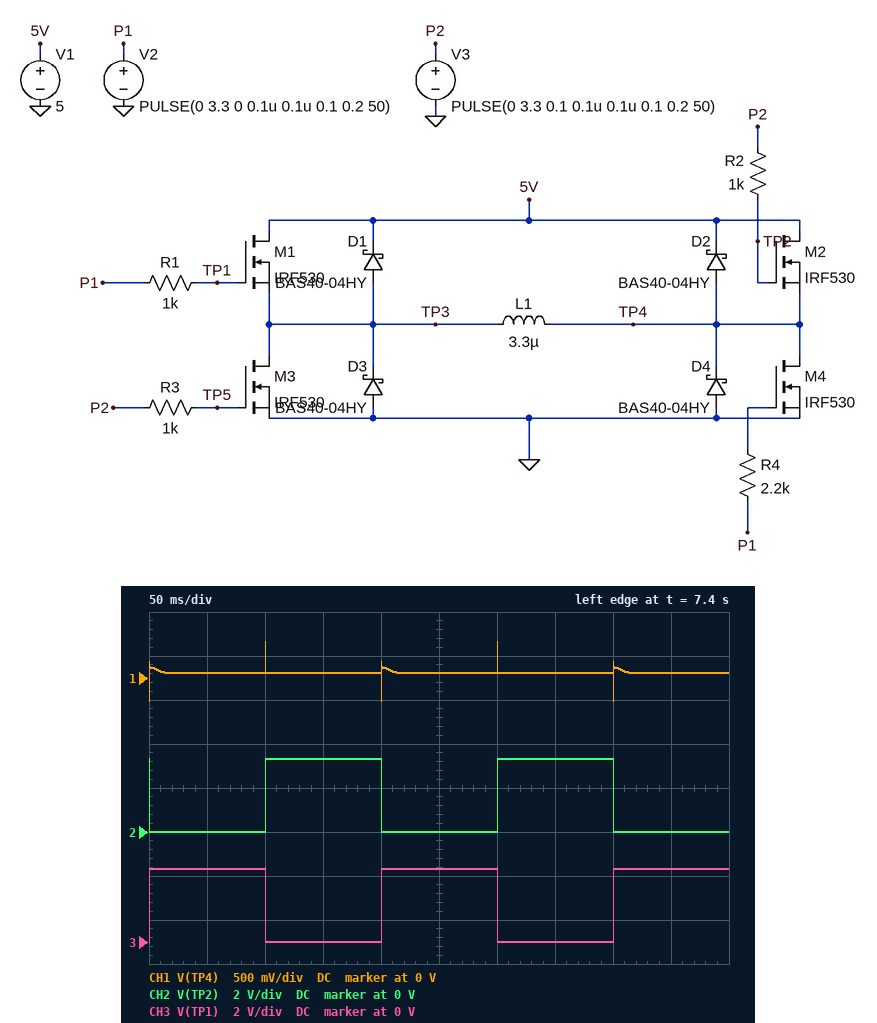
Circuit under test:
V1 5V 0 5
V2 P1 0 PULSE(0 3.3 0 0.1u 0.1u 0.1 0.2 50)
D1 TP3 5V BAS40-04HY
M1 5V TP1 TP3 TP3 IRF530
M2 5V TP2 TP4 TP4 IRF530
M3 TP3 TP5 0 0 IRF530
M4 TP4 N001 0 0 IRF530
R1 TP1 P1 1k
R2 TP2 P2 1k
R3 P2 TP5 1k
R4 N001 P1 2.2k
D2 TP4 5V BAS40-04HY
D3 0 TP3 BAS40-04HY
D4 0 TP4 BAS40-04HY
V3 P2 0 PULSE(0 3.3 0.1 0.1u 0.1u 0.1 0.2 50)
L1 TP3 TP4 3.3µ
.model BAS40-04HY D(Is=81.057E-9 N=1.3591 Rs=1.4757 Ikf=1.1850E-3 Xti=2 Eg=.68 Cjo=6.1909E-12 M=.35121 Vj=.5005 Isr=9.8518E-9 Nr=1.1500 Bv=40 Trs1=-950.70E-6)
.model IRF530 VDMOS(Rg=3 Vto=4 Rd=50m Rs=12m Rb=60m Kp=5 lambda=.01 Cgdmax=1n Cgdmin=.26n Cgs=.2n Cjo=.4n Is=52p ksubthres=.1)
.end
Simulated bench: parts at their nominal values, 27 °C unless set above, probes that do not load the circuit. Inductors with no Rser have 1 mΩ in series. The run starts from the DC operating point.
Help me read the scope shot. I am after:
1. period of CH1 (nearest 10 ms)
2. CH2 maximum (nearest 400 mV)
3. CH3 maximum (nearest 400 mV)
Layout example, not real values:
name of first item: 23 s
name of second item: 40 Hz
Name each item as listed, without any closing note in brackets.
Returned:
period of CH1: 200 ms
CH2 maximum: 3.2 V
CH3 maximum: 3.2 V
